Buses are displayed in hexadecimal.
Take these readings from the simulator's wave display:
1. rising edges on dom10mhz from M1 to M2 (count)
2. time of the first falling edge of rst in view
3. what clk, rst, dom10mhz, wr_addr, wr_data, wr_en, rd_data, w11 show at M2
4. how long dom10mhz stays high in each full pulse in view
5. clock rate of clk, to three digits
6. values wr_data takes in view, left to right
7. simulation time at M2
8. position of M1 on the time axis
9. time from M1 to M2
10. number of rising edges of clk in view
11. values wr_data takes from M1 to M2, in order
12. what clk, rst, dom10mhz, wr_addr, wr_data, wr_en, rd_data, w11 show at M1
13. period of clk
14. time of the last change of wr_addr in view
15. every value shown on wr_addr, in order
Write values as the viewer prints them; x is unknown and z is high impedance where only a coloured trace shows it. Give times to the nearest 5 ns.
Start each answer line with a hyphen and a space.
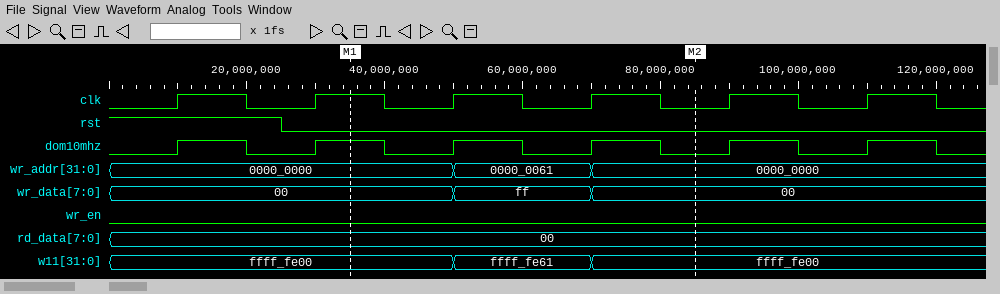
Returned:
- 2
- 25 ns
- clk=0, rst=0, dom10mhz=0, wr_addr=0000_0000, wr_data=00, wr_en=0, rd_data=00, w11=ffff_fe00
- 10 ns, 10 ns, 10 ns, 10 ns, 10 ns, 10 ns
- 50.0 MHz
- 00, ff, 00
- 85 ns
- 35 ns
- 50 ns
- 6
- 00, ff, 00
- clk=1, rst=0, dom10mhz=1, wr_addr=0000_0000, wr_data=00, wr_en=0, rd_data=00, w11=ffff_fe00
- 20 ns
- 70 ns
- 0000_0000, 0000_0061, 0000_0000
